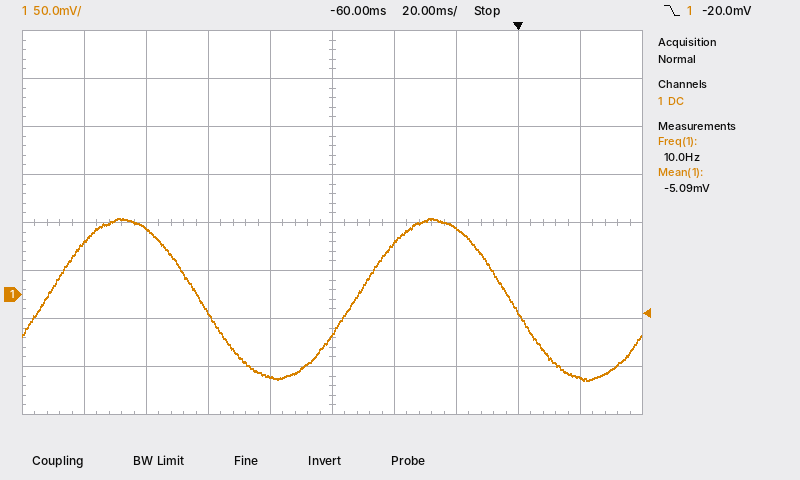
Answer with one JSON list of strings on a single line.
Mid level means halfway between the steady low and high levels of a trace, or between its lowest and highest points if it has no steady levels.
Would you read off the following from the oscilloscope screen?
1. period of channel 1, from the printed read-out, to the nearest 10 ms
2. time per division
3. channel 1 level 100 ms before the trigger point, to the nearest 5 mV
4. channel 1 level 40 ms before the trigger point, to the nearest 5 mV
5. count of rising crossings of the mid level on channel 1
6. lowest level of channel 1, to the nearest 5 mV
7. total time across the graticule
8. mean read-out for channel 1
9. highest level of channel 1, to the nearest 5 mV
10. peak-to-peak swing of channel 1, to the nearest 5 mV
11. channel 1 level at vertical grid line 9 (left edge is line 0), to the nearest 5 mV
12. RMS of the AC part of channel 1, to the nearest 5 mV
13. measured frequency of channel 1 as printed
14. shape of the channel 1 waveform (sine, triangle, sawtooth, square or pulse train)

["100 ms", "20 ms", "-20 mV", "55 mV", "2", "-90 mV", "200 ms", "-5.09 mV", "80 mV", "170 mV", "-85 mV", "60 mV", "10.0 Hz", "sine"]
